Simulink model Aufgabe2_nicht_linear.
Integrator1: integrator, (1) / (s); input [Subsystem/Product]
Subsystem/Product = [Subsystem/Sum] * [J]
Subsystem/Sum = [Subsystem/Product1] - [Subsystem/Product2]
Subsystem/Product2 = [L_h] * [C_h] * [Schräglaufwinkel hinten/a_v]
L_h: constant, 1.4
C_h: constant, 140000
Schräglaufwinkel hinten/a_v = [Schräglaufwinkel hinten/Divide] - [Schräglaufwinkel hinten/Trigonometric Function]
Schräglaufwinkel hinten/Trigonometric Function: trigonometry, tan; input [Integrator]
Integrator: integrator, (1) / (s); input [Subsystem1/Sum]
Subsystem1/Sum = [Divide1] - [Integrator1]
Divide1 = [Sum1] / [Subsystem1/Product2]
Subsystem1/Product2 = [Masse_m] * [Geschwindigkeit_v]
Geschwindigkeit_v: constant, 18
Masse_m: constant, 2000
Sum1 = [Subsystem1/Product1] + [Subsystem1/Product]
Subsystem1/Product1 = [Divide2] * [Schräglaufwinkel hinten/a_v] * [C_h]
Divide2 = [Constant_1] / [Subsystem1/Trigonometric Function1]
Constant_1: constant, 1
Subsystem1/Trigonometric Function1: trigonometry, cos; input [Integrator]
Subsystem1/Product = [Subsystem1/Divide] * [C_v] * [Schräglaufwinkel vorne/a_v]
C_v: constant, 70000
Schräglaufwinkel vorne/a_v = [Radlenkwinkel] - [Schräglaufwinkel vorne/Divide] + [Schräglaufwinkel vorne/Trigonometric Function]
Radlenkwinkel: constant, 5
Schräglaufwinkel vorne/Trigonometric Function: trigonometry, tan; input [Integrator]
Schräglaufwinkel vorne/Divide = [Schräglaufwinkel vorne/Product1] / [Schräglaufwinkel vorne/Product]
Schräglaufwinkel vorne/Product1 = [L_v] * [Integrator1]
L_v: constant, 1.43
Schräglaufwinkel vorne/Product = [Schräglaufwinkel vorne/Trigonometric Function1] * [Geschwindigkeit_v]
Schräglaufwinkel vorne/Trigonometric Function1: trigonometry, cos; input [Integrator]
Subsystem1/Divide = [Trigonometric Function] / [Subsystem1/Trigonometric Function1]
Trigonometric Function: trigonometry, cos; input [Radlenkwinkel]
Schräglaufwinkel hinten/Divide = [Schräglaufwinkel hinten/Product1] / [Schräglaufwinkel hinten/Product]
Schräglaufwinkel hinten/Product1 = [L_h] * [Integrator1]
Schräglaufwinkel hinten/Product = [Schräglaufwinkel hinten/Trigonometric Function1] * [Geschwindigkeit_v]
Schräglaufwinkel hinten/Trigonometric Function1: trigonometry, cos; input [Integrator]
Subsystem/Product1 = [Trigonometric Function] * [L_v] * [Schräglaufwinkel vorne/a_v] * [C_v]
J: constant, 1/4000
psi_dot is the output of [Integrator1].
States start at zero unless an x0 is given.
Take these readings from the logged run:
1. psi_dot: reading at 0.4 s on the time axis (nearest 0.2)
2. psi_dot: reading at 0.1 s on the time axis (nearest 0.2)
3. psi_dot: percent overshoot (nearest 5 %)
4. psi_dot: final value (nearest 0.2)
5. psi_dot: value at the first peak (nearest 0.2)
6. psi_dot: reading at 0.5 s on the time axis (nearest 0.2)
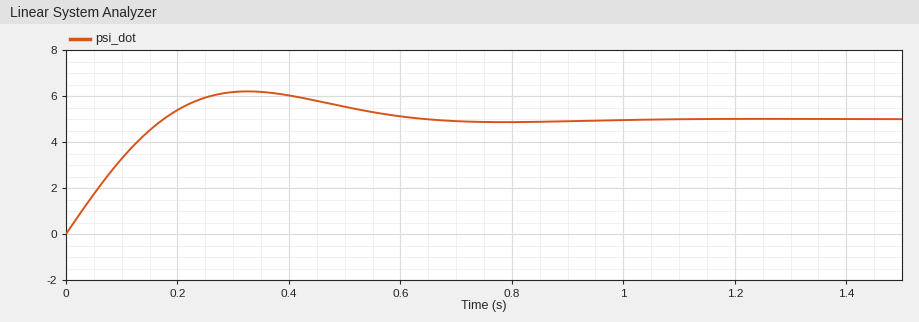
6.0
3.2
25 %
5.0
6.2
5.6
